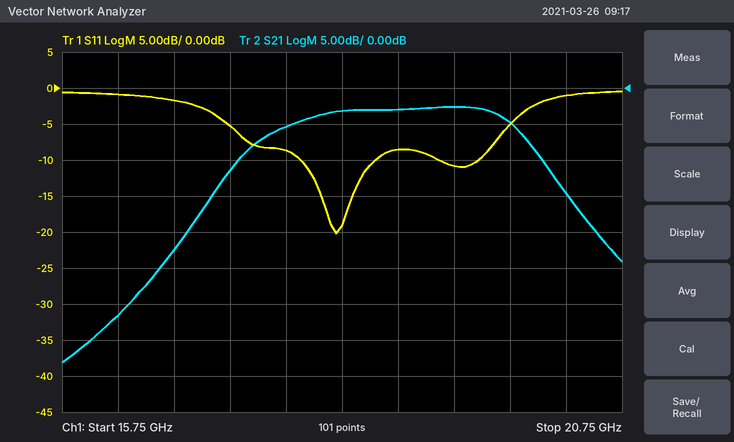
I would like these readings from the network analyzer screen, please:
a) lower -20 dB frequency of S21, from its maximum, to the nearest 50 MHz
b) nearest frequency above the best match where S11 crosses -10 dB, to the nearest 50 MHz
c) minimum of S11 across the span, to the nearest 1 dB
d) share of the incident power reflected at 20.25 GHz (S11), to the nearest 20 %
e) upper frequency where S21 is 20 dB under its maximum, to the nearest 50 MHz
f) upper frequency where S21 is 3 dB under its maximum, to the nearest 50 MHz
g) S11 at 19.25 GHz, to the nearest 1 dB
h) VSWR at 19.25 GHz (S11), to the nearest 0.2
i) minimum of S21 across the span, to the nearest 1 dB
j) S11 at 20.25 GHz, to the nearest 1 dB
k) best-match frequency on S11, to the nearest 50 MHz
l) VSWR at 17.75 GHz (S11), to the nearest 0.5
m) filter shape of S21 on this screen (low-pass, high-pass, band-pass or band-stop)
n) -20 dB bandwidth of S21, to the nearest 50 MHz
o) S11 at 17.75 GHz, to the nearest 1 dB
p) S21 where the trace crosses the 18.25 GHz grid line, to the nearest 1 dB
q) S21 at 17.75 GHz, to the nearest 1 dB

16.75 GHz
18.55 GHz
-20 dB
80 %
20.65 GHz
19.80 GHz
-11 dB
1.8
-38 dB
-1 dB
18.20 GHz
2.0
band-pass
3.90 GHz
-9 dB
-3 dB
-5 dB
